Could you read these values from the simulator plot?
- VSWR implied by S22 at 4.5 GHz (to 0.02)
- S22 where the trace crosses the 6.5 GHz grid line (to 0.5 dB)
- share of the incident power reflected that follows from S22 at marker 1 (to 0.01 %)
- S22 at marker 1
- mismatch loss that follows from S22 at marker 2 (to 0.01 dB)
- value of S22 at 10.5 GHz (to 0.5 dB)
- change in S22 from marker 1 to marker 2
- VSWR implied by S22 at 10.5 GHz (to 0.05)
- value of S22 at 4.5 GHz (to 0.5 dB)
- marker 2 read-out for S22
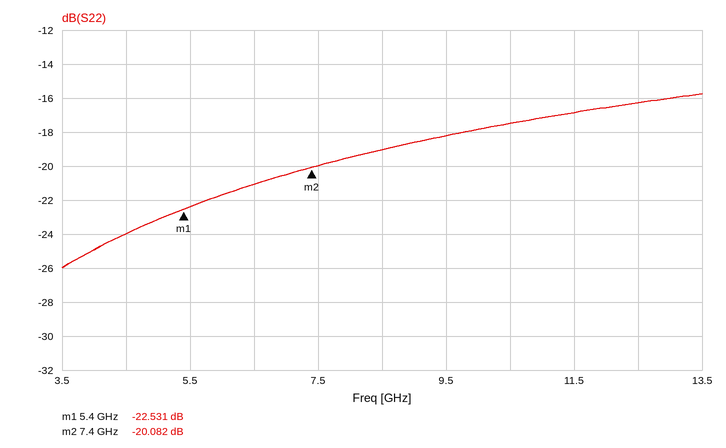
1.14
-21.0 dB
0.56 %
-22.531 dB
0.04 dB
-17.5 dB
2.449 dB
1.30
-24.0 dB
-20.082 dB
